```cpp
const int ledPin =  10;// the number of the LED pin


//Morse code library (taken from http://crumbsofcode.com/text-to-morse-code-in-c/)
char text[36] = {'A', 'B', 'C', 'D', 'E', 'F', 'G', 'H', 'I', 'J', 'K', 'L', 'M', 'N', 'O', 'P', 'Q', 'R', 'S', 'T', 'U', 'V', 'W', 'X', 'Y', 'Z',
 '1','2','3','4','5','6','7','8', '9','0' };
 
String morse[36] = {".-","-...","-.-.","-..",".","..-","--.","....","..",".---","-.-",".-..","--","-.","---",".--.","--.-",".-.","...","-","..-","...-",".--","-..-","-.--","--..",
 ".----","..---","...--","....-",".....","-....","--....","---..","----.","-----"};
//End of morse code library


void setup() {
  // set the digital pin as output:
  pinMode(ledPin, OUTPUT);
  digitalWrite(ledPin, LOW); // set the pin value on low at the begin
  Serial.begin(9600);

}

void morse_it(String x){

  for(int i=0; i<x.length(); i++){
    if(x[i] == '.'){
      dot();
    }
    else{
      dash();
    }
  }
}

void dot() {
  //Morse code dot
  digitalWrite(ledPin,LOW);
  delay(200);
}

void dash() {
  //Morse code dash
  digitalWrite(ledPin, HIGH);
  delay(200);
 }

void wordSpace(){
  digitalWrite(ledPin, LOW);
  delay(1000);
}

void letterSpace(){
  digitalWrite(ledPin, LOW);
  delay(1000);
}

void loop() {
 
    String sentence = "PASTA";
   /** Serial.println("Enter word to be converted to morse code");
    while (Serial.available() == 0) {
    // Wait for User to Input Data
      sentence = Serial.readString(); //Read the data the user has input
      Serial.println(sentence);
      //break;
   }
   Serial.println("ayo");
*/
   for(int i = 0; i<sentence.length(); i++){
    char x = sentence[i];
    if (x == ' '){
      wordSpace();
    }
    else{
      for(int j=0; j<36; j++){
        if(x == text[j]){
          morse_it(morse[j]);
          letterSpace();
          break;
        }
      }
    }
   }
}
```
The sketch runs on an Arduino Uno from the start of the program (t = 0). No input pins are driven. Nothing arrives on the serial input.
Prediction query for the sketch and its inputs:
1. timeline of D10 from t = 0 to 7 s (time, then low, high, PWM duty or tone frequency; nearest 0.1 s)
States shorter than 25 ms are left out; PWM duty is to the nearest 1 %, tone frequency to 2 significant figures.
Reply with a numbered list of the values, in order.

1. 0 s low; 0.2 s high; 0.6 s low; 2 s high; 2.2 s low; 4.8 s high; 5 s low; 6.2 s high; 6.4 s low
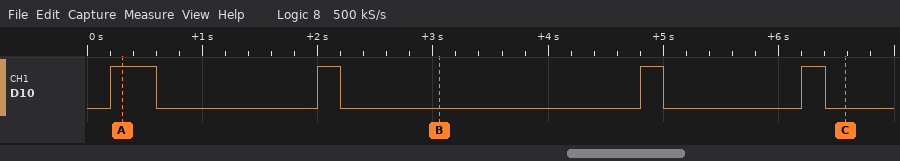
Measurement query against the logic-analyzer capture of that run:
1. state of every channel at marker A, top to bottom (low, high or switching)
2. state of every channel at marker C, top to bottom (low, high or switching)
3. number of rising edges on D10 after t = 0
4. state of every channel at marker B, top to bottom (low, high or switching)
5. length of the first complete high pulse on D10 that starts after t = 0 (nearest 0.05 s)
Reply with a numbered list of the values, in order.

1. D10 high
2. D10 low
3. 4
4. D10 low
5. 0.40 s
